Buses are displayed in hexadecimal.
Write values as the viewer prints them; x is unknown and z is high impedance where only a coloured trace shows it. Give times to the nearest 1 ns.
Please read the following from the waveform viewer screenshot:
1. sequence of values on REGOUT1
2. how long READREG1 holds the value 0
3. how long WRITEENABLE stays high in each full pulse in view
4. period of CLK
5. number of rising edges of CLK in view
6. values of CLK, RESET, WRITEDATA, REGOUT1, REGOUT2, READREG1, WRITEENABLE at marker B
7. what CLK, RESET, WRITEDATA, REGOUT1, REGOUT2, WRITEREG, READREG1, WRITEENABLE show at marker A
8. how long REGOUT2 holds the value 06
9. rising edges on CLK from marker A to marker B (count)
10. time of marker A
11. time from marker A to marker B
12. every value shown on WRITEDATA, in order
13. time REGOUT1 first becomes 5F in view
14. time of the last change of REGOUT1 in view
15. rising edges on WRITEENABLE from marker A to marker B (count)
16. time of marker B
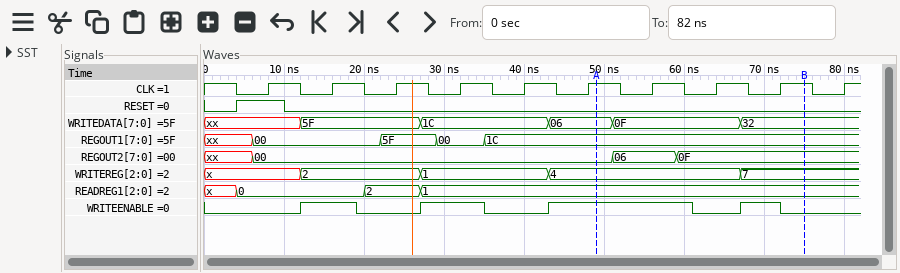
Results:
xx, 00, 5F, 00, 1C
16 ns
7 ns, 8 ns, 18 ns, 5 ns
8 ns
10
CLK=1, RESET=0, WRITEDATA=32, REGOUT1=1C, REGOUT2=0F, READREG1=1, WRITEENABLE=0
CLK=1, RESET=0, WRITEDATA=06, REGOUT1=1C, REGOUT2=00, WRITEREG=4, READREG1=1, WRITEENABLE=1
8 ns
3
49 ns
26 ns
xx, 5F, 1C, 06, 0F, 32
22 ns
35 ns
1
75 ns
